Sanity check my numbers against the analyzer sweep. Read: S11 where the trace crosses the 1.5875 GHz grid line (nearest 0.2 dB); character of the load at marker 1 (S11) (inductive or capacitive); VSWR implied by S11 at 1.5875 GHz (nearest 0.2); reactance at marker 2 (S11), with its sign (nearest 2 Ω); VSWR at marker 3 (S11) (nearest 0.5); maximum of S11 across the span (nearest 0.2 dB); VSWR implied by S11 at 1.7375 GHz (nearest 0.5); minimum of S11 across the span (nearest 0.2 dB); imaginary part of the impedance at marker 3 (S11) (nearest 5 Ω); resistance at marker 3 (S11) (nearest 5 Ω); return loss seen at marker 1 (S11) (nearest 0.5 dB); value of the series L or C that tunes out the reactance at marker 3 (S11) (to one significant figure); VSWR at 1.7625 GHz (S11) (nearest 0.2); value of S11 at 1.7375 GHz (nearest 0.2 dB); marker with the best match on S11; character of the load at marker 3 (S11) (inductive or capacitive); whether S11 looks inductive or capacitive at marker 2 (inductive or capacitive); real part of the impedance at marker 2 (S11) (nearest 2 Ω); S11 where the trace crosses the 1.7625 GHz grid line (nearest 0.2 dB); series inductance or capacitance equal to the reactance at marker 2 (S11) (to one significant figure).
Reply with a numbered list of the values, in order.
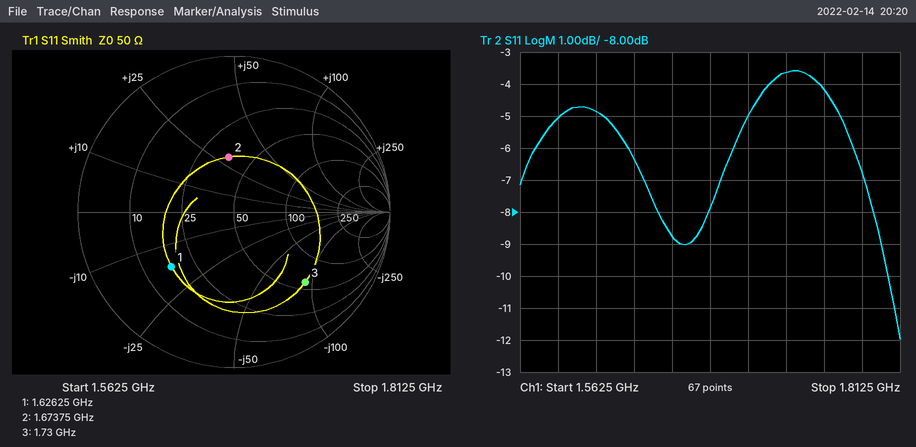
1. -5.0 dB
2. capacitive
3. 3.6
4. +30 Ω
5. 4.5
6. -3.6 dB
7. 5.0
8. -12.0 dB
9. -90 Ω
10. 60 Ω
11. 5.5 dB
12. 8 nH
13. 4.2
14. -3.6 dB
15. marker 2
16. capacitive
17. inductive
18. 36 Ω
19. -4.2 dB
20. 3 nH
